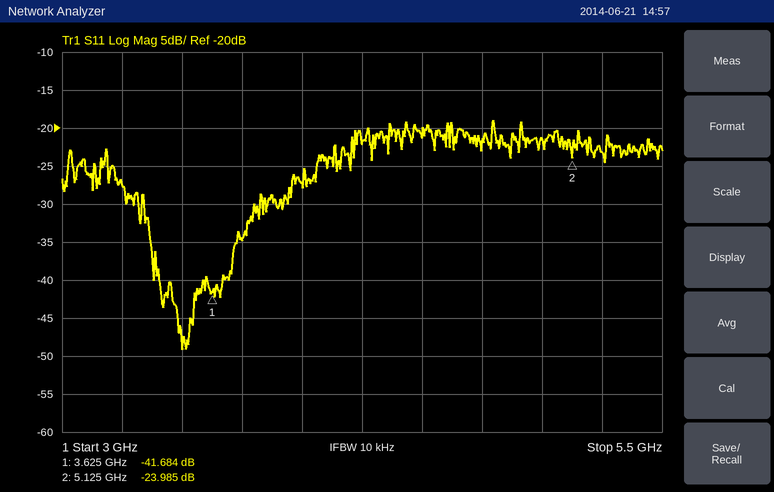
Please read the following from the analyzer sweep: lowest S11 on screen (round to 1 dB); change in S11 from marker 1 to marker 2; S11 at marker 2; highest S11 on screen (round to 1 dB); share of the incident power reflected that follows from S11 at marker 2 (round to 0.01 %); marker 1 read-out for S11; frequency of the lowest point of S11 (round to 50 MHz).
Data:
-49 dB
17.699 dB
-23.985 dB
-19 dB
0.40 %
-41.684 dB
3.50 GHz
